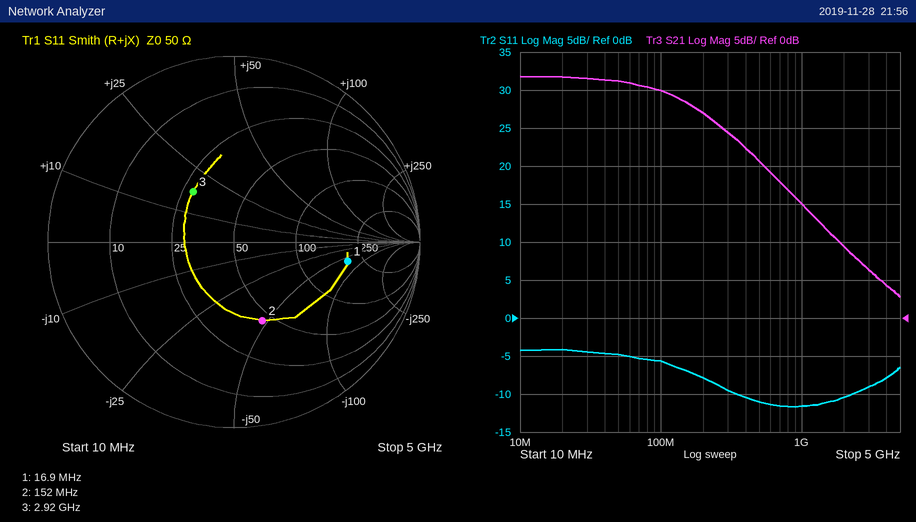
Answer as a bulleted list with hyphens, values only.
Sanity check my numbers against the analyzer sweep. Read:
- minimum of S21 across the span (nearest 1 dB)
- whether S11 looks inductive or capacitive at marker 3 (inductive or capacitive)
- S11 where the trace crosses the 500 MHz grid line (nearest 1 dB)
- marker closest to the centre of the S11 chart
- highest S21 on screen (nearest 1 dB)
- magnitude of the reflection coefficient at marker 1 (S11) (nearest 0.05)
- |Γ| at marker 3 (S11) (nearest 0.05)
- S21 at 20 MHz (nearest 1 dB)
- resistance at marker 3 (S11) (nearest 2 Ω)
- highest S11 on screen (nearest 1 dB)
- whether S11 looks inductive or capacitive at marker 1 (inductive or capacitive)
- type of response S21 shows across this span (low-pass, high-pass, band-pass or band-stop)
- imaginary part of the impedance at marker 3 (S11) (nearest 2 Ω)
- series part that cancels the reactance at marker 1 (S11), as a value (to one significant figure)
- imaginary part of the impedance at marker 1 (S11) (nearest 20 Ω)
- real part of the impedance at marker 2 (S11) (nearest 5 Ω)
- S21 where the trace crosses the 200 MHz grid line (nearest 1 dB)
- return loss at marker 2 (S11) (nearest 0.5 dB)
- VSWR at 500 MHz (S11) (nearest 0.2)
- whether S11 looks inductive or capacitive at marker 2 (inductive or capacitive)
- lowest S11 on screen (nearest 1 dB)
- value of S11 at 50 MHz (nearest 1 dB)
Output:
- 3 dB
- inductive
- -11 dB
- marker 3
- 32 dB
- 0.60
- 0.35
- 32 dB
- 28 Ω
- -4 dB
- capacitive
- low-pass
- +18 Ω
- 600 nH
- -60 Ω
- 45 Ω
- 27 dB
- 7.0 dB
- 1.8
- capacitive
- -12 dB
- -5 dB
